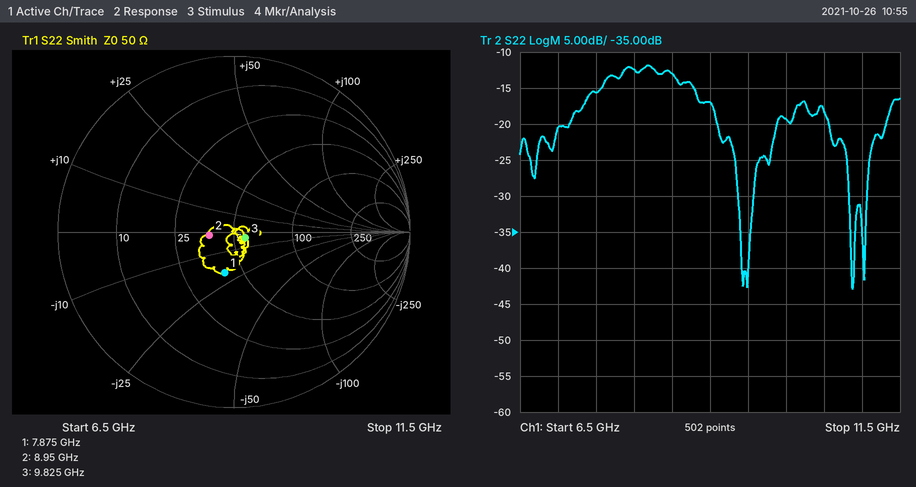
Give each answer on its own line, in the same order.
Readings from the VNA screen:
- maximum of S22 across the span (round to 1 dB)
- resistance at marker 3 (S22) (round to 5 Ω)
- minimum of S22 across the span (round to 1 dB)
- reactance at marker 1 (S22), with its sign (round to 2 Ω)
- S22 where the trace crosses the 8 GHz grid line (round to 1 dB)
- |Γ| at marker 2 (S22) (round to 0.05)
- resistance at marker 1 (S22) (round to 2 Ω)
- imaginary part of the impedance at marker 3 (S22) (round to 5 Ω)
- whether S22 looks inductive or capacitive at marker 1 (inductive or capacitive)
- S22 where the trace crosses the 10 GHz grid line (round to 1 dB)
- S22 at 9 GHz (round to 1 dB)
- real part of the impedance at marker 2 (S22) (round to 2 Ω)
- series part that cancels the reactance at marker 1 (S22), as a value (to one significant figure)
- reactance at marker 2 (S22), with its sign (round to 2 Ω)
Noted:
-12 dB
55 Ω
-43 dB
-20 Ω
-12 dB
0.15
40 Ω
-5 Ω
capacitive
-19 dB
-17 dB
38 Ω
400 pH
-2 Ω
